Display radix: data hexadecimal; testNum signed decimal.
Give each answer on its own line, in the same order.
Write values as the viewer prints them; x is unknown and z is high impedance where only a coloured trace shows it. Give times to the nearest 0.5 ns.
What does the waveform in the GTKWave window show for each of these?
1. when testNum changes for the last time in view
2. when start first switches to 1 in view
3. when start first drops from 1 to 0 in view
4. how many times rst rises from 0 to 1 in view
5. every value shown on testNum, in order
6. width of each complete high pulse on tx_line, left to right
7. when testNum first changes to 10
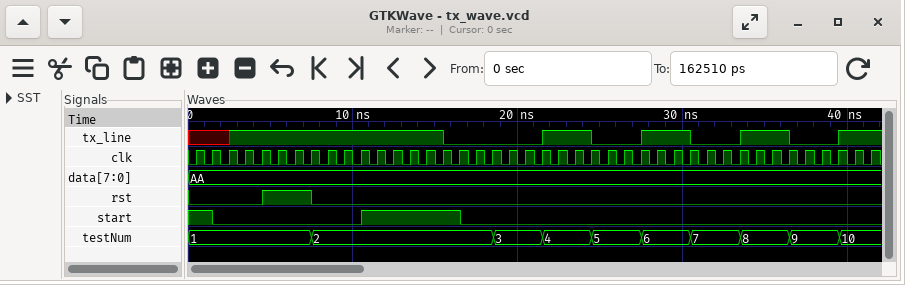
39.5 ns
10.5 ns
1.5 ns
1
1, 2, 3, 4, 5, 6, 7, 8, 9, 10
3 ns, 3 ns, 3 ns
39.5 ns
